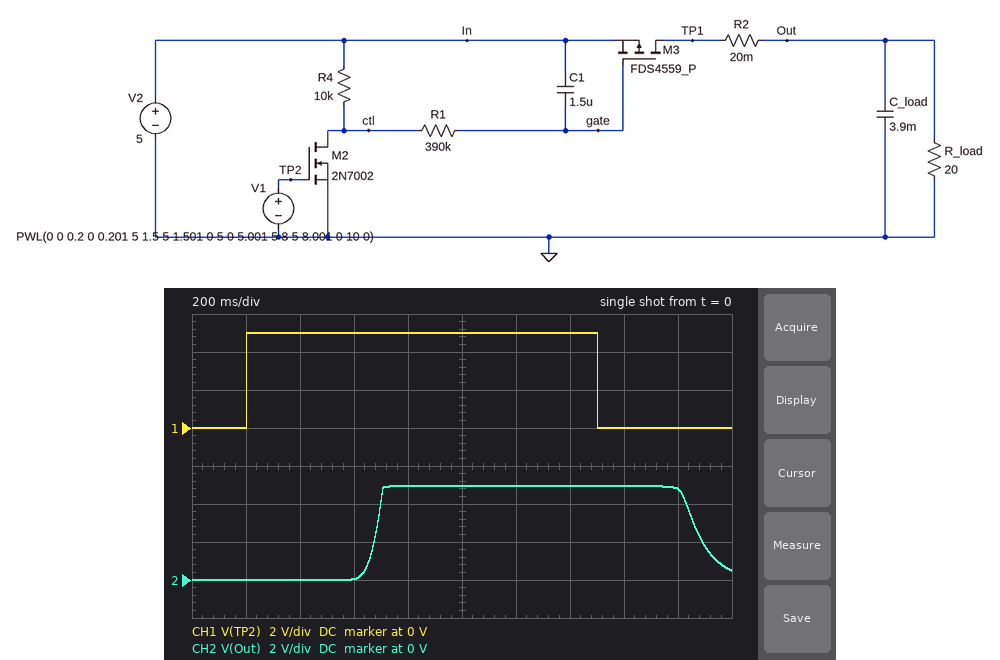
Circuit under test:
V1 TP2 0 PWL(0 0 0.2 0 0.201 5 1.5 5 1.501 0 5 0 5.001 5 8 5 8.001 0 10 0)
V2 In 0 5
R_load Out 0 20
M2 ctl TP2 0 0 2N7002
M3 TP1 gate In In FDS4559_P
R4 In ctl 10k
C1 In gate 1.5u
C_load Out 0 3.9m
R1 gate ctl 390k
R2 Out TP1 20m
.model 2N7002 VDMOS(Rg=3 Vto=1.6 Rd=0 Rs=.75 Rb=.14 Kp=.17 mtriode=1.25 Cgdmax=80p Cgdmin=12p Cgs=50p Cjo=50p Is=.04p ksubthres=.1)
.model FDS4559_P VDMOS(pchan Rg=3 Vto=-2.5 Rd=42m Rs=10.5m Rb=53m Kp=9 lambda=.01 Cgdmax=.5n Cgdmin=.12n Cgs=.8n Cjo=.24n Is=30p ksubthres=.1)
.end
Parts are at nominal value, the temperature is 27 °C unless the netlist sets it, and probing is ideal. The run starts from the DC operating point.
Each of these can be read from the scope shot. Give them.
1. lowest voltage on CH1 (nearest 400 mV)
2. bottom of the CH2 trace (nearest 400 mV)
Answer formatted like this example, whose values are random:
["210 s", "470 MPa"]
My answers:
["0 V", "0 V"]
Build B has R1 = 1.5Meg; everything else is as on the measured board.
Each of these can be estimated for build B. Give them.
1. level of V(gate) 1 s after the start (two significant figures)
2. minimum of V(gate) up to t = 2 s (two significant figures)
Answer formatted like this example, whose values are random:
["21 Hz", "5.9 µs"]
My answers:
["3.5 V", "2.8 V"]
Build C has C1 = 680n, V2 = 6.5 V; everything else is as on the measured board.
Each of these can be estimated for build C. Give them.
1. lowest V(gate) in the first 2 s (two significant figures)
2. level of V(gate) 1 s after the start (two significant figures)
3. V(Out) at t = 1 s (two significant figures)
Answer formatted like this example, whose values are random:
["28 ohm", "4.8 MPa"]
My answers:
["50 mV", "320 mV", "6.5 V"]
